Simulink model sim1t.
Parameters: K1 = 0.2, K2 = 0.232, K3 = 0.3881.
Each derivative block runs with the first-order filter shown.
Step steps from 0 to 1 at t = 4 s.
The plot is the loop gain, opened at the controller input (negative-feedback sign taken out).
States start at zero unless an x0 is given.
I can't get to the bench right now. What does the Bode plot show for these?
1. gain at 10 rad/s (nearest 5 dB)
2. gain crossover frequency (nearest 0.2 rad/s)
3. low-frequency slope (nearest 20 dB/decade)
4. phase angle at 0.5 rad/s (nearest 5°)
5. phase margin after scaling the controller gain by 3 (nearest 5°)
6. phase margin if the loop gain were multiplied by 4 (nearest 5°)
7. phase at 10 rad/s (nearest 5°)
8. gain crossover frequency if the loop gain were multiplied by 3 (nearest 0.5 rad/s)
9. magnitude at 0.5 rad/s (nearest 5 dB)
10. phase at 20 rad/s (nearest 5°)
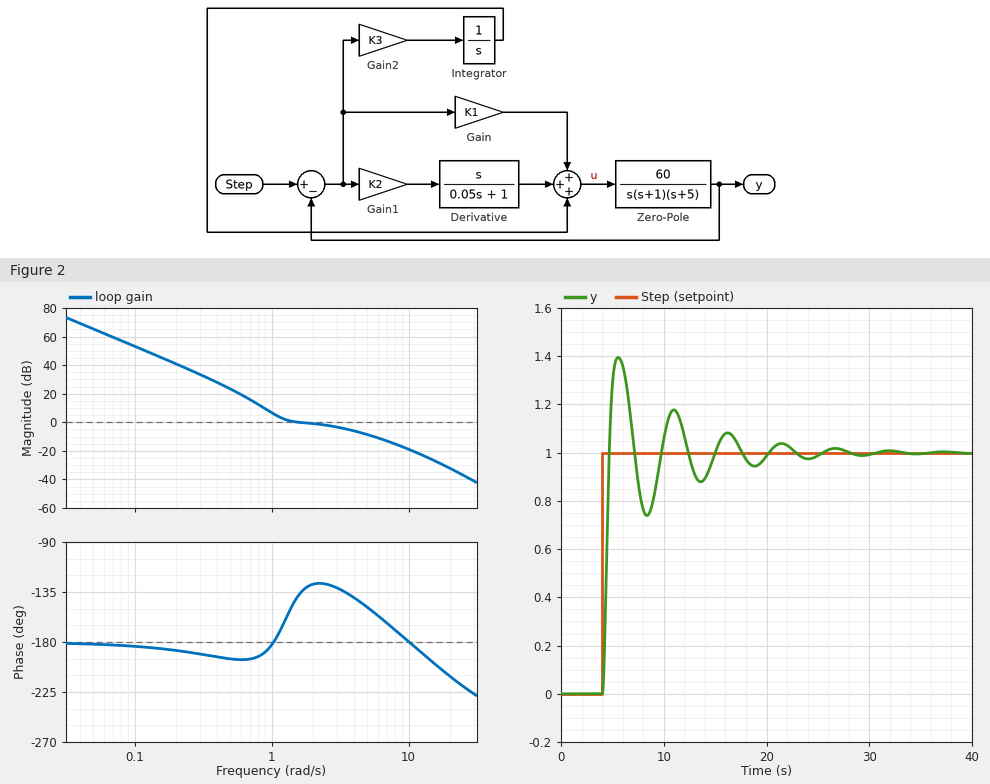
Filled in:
-20 dB
1.6 rad/s
-40 dB/decade
-195°
30°
20°
-180°
5.5 rad/s
25 dB
-210°
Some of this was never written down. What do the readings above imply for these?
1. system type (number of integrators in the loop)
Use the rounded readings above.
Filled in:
2
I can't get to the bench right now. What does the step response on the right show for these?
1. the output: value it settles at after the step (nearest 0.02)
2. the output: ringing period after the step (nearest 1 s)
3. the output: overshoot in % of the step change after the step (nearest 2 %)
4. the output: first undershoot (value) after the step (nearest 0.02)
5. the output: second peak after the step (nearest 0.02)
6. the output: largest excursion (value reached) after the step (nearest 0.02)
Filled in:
1.00
5 s
40 %
0.74
1.18
1.40
